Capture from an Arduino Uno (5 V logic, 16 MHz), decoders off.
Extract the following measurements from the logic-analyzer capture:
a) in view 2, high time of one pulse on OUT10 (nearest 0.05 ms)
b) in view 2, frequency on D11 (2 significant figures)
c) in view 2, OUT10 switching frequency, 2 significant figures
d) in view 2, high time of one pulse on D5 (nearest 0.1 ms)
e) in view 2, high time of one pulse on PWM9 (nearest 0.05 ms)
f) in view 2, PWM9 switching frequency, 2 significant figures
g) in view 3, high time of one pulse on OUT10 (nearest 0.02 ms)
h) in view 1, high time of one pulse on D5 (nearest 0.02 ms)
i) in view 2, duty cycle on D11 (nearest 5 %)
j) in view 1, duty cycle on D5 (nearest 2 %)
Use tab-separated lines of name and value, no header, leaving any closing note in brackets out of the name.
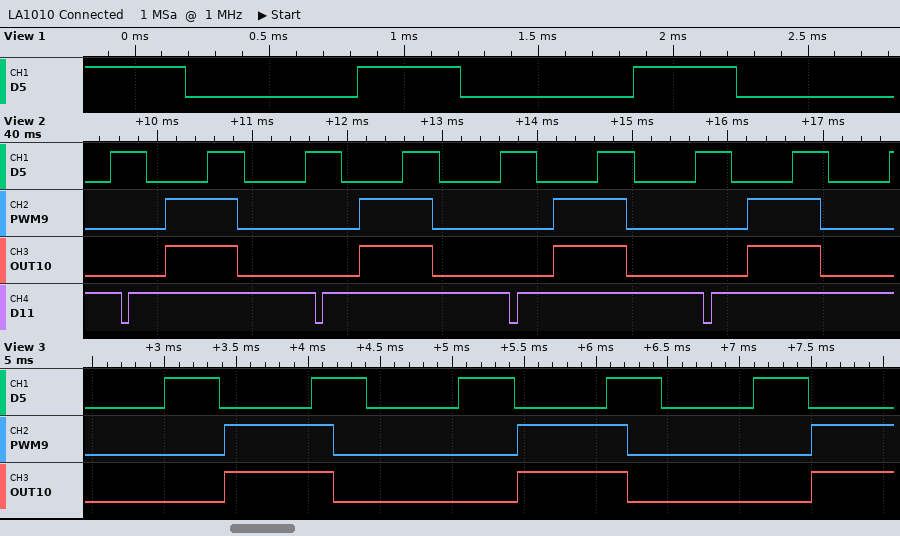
in view 2, high time of one pulse on OUT10	0.75 ms
in view 2, frequency on D11	490 Hz
in view 2, OUT10 switching frequency, 2 significant figures	490 Hz
in view 2, high time of one pulse on D5	0.4 ms
in view 2, high time of one pulse on PWM9	0.75 ms
in view 2, PWM9 switching frequency, 2 significant figures	490 Hz
in view 3, high time of one pulse on OUT10	0.76 ms
in view 1, high time of one pulse on D5	0.38 ms
in view 2, duty cycle on D11	95 %
in view 1, duty cycle on D5	38 %
